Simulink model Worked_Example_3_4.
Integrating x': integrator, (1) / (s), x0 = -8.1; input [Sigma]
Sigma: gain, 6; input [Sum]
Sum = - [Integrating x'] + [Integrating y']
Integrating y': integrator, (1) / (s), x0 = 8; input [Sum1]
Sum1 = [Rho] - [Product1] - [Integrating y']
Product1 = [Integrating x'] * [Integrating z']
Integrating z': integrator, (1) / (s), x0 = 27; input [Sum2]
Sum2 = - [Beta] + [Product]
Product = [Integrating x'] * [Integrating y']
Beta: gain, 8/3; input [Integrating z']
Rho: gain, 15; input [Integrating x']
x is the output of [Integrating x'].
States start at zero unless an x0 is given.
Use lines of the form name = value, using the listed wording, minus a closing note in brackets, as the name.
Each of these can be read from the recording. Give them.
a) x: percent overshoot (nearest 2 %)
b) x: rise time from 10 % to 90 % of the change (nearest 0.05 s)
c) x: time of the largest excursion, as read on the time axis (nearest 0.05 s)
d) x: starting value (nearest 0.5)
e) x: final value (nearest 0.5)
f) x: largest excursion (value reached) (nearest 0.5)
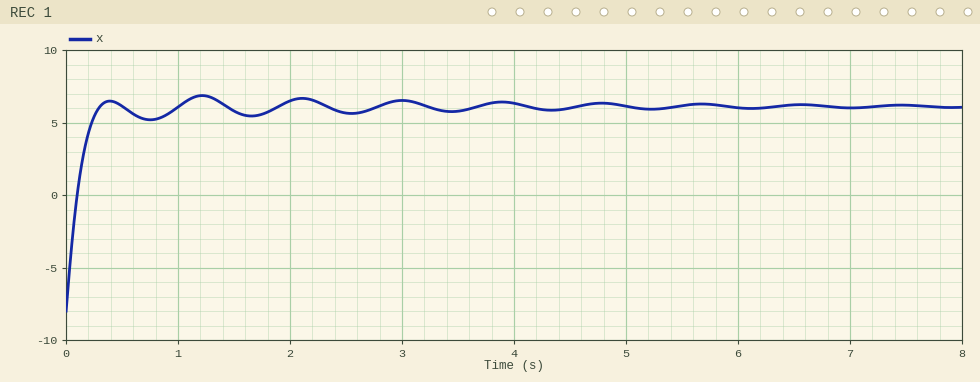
x: percent overshoot = 6 %
x: rise time from 10 % to 90 % of the change = 0.20 s
x: time of the largest excursion, as read on the time axis = 1.20 s
x: starting value = -8.0
x: final value = 6.0
x: largest excursion (value reached) = 7.0
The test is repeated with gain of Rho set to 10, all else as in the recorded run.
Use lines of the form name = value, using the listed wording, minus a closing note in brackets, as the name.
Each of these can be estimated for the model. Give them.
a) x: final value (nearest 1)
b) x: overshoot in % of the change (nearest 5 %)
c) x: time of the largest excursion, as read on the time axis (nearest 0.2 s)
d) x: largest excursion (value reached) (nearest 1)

x: final value = 5
x: overshoot in % of the change = 15 %
x: time of the largest excursion, as read on the time axis = 1.4 s
x: largest excursion (value reached) = 7
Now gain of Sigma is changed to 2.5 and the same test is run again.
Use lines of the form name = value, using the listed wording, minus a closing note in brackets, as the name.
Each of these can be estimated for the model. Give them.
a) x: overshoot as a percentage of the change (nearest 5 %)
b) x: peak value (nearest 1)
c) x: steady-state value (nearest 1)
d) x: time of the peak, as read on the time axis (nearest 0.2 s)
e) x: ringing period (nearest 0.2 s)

x: overshoot as a percentage of the change = 10 %
x: peak value = 8
x: steady-state value = 6
x: time of the peak, as read on the time axis = 0.8 s
x: ringing period = 1.0 s
